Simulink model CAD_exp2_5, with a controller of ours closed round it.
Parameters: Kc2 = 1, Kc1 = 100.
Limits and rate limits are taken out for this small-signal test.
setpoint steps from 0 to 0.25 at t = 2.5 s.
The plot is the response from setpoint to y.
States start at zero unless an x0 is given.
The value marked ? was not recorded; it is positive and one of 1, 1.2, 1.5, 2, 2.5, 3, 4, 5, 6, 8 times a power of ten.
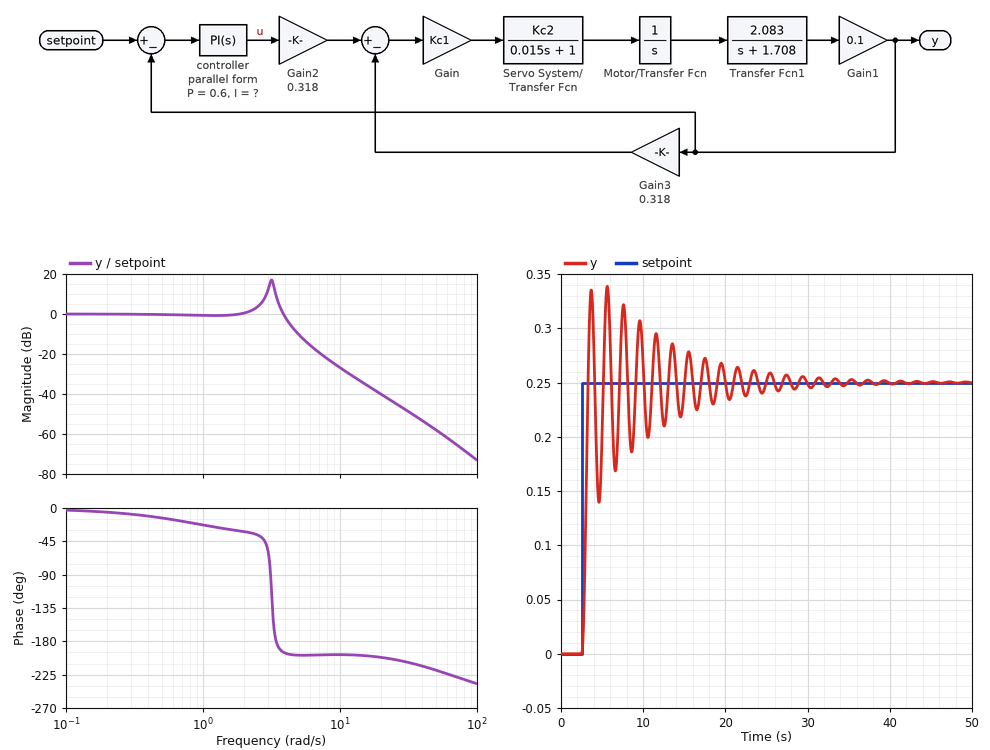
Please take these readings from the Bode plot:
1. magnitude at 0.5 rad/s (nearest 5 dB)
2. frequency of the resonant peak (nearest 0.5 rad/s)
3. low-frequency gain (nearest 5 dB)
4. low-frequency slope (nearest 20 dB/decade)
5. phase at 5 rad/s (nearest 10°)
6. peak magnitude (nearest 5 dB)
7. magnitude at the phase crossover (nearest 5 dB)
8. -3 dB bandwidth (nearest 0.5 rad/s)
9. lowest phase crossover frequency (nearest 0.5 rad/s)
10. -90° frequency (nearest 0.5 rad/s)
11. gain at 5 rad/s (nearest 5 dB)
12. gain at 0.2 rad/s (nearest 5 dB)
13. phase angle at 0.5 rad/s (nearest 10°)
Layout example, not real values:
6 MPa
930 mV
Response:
0 dB
3.0 rad/s
0 dB
0 dB/decade
-200°
15 dB
10 dB
4.0 rad/s
3.5 rad/s
3.0 rad/s
-10 dB
0 dB
-10°
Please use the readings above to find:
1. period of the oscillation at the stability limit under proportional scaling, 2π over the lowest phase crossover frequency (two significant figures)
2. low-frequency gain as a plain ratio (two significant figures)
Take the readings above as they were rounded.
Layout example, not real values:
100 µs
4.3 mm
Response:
1.8 s
1.0
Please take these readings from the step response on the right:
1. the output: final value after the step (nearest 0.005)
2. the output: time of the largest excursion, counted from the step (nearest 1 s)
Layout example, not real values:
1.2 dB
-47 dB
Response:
0.250
3 s
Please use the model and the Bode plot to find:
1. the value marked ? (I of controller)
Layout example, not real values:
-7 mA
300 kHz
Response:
2
